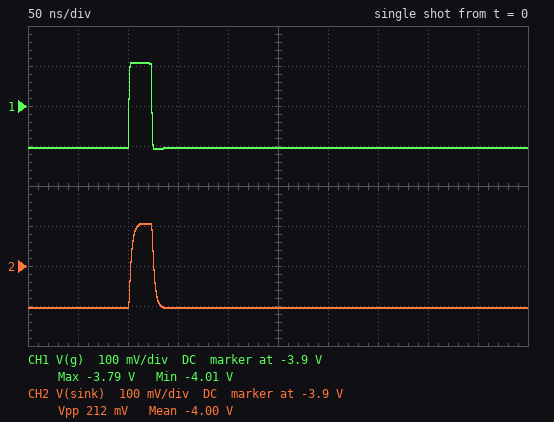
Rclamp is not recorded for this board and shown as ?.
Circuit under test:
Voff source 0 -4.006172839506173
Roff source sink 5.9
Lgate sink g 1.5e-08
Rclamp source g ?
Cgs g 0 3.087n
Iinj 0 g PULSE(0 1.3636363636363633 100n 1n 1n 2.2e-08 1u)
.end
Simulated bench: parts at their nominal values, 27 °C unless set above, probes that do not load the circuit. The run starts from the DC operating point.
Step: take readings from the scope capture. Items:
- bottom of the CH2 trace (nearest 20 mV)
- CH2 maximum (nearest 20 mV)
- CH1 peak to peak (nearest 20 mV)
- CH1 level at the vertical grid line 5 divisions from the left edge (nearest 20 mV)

-4.00 V
-3.80 V
220 mV
-4.00 V
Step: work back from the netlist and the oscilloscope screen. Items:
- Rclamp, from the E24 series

0.16 Ω
